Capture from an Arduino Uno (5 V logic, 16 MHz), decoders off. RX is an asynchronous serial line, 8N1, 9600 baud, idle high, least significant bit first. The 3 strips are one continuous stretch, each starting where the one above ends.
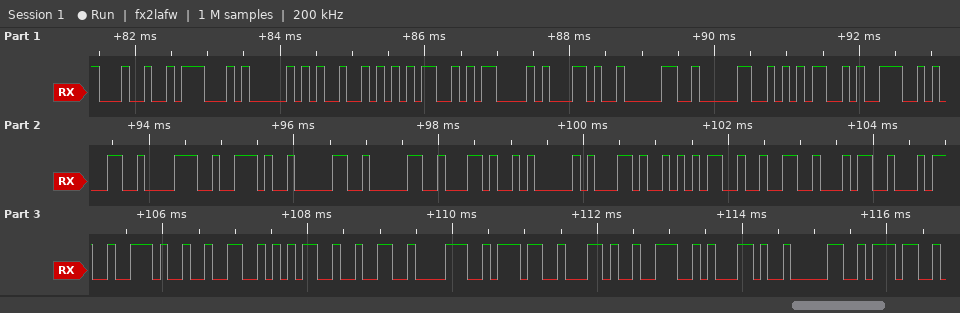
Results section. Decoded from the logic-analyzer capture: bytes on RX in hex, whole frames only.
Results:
24 47 50 52 4D 43 2C 30 30 35 39 31 38 2E 30 30 2C 41 2C 35 32 34 34 2E 32 35 32 38 37 2C 4E 2C 30 37
